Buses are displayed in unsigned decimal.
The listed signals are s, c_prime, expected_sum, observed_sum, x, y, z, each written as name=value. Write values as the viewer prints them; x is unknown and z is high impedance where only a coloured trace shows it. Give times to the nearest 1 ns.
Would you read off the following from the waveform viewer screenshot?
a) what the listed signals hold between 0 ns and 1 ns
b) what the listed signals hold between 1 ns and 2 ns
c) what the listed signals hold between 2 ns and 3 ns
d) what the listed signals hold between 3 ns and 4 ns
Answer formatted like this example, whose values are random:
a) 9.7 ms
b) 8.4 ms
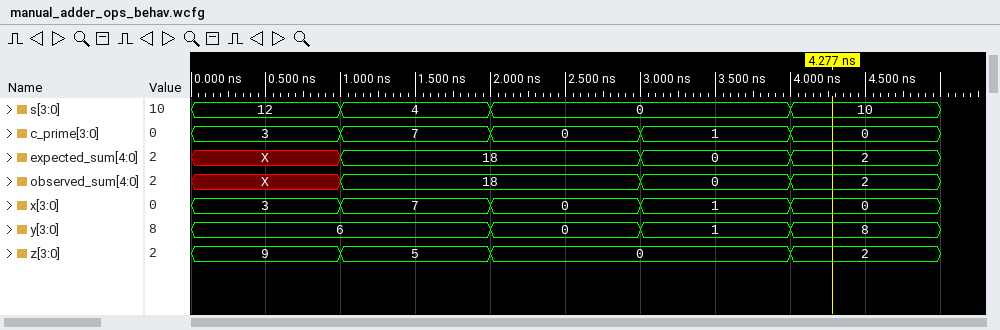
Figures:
a) s=12, c_prime=3, expected_sum=X, observed_sum=X, x=3, y=6, z=9
b) s=4, c_prime=7, expected_sum=18, observed_sum=18, x=7, y=6, z=5
c) s=0, c_prime=0, expected_sum=18, observed_sum=18, x=0, y=0, z=0
d) s=0, c_prime=1, expected_sum=0, observed_sum=0, x=1, y=1, z=0
